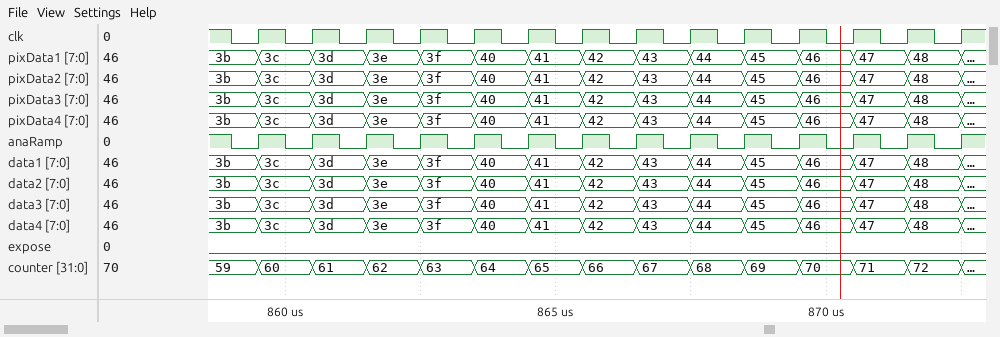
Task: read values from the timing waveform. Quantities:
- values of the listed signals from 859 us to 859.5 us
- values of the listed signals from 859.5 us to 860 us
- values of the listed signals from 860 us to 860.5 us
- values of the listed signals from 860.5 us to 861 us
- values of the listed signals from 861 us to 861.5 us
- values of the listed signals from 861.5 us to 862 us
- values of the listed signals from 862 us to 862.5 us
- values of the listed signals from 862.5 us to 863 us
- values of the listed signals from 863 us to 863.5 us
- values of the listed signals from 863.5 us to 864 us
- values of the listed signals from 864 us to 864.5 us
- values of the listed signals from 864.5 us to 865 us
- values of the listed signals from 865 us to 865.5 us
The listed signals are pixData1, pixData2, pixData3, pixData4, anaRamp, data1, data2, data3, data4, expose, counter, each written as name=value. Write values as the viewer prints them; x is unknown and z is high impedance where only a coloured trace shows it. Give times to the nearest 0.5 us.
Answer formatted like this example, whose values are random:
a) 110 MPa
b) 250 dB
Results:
a) pixData1=3b, pixData2=3b, pixData3=3b, pixData4=3b, anaRamp=0, data1=3b, data2=3b, data3=3b, data4=3b, expose=0, counter=59
b) pixData1=3c, pixData2=3c, pixData3=3c, pixData4=3c, anaRamp=1, data1=3c, data2=3c, data3=3c, data4=3c, expose=0, counter=60
c) pixData1=3c, pixData2=3c, pixData3=3c, pixData4=3c, anaRamp=0, data1=3c, data2=3c, data3=3c, data4=3c, expose=0, counter=60
d) pixData1=3d, pixData2=3d, pixData3=3d, pixData4=3d, anaRamp=1, data1=3d, data2=3d, data3=3d, data4=3d, expose=0, counter=61
e) pixData1=3d, pixData2=3d, pixData3=3d, pixData4=3d, anaRamp=0, data1=3d, data2=3d, data3=3d, data4=3d, expose=0, counter=61
f) pixData1=3e, pixData2=3e, pixData3=3e, pixData4=3e, anaRamp=1, data1=3e, data2=3e, data3=3e, data4=3e, expose=0, counter=62
g) pixData1=3e, pixData2=3e, pixData3=3e, pixData4=3e, anaRamp=0, data1=3e, data2=3e, data3=3e, data4=3e, expose=0, counter=62
h) pixData1=3f, pixData2=3f, pixData3=3f, pixData4=3f, anaRamp=1, data1=3f, data2=3f, data3=3f, data4=3f, expose=0, counter=63
i) pixData1=3f, pixData2=3f, pixData3=3f, pixData4=3f, anaRamp=0, data1=3f, data2=3f, data3=3f, data4=3f, expose=0, counter=63
j) pixData1=40, pixData2=40, pixData3=40, pixData4=40, anaRamp=1, data1=40, data2=40, data3=40, data4=40, expose=0, counter=64
k) pixData1=40, pixData2=40, pixData3=40, pixData4=40, anaRamp=0, data1=40, data2=40, data3=40, data4=40, expose=0, counter=64
l) pixData1=41, pixData2=41, pixData3=41, pixData4=41, anaRamp=1, data1=41, data2=41, data3=41, data4=41, expose=0, counter=65
m) pixData1=41, pixData2=41, pixData3=41, pixData4=41, anaRamp=0, data1=41, data2=41, data3=41, data4=41, expose=0, counter=65
